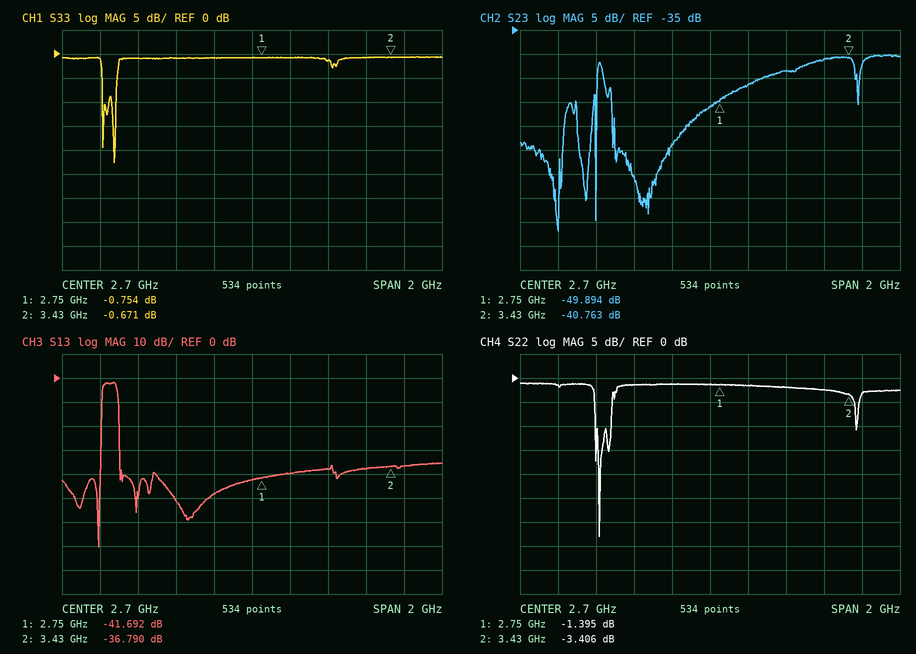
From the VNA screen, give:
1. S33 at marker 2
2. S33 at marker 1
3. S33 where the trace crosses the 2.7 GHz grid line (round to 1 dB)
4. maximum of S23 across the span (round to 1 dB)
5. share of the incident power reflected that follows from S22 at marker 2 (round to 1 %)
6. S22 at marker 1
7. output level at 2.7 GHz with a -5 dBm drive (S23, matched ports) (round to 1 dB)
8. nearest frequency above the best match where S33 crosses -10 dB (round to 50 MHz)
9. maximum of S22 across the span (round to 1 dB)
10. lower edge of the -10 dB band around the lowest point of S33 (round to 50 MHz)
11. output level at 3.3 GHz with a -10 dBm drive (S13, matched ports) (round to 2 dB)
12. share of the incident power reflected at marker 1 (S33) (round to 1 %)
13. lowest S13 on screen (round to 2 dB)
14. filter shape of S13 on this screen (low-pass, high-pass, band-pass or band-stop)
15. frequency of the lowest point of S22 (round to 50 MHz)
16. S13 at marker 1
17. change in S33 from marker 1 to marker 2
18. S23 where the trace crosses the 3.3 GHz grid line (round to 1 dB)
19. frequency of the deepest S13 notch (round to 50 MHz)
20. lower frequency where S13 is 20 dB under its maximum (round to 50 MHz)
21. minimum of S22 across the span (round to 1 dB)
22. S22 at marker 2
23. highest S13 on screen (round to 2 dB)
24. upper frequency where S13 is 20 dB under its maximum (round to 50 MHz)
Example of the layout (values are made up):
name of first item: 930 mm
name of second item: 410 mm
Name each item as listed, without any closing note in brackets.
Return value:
S33 at marker 2: -0.671 dB
S33 at marker 1: -0.754 dB
S33 where the trace crosses the 2.7 GHz grid line: -1 dB
maximum of S23 across the span: -40 dB
share of the incident power reflected that follows from S22 at marker 2: 46 %
S22 at marker 1: -1.395 dB
output level at 2.7 GHz with a -5 dBm drive (S23, matched ports): -56 dBm
nearest frequency above the best match where S33 crosses -10 dB: 2.00 GHz
maximum of S22 across the span: -1 dB
lower edge of the -10 dB band around the lowest point of S33: 1.95 GHz
output level at 3.3 GHz with a -10 dBm drive (S13, matched ports): -48 dBm
share of the incident power reflected at marker 1 (S33): 84 %
lowest S13 on screen: -70 dB
filter shape of S13 on this screen: band-pass
frequency of the lowest point of S22: 2.10 GHz
S13 at marker 1: -41.692 dB
change in S33 from marker 1 to marker 2: 0.083 dB
S23 where the trace crosses the 3.3 GHz grid line: -41 dB
frequency of the deepest S13 notch: 1.90 GHz
lower frequency where S13 is 20 dB under its maximum: 1.90 GHz
minimum of S22 across the span: -33 dB
S22 at marker 2: -3.406 dB
highest S13 on screen: -2 dB
upper frequency where S13 is 20 dB under its maximum: 2.00 GHz
